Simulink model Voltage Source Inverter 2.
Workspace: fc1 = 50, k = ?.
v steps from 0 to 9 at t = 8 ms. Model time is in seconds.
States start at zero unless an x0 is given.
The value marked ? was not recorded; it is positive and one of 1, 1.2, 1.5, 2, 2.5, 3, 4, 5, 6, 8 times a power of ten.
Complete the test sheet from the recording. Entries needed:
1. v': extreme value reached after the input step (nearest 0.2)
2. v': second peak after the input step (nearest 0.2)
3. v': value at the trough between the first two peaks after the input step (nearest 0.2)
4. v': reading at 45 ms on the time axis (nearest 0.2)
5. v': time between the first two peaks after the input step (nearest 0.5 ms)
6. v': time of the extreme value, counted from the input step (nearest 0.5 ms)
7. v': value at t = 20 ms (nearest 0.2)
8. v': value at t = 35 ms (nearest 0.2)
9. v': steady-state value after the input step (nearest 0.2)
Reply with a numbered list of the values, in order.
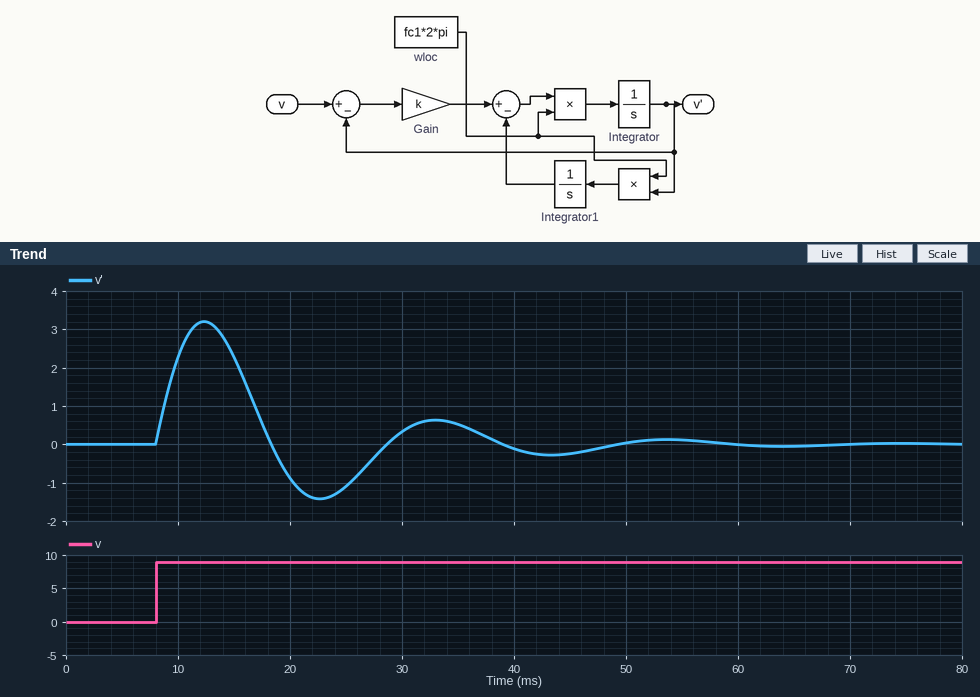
1. 3.2
2. 0.6
3. -1.4
4. -0.2
5. 20.5 ms
6. 4.5 ms
7. -0.8
8. 0.6
9. 0.0
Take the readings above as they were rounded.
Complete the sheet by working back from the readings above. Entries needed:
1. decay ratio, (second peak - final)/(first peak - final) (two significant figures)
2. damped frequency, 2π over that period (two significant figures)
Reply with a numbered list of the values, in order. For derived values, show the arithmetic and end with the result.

1. (0.6 - 0) / (3.2 - 0) = 0.19
2. 2π / 20.5 = 0.31 rad/ms
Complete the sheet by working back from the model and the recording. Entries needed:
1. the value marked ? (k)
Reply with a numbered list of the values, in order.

1. 0.5
